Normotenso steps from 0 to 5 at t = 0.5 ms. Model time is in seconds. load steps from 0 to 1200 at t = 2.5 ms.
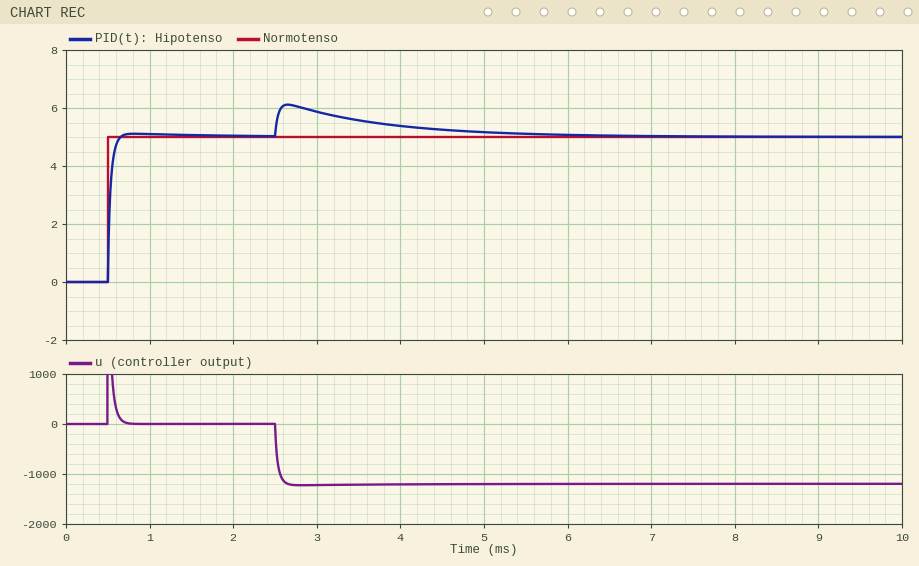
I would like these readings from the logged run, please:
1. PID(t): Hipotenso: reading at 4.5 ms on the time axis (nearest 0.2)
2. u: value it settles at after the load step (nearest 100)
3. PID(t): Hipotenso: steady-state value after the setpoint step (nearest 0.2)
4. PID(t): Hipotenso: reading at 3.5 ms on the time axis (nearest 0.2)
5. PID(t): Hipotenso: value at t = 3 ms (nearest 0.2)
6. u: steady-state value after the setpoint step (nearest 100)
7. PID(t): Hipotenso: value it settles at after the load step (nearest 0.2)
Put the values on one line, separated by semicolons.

5.2; -1200; 5.0; 5.6; 5.8; 0; 5.0
